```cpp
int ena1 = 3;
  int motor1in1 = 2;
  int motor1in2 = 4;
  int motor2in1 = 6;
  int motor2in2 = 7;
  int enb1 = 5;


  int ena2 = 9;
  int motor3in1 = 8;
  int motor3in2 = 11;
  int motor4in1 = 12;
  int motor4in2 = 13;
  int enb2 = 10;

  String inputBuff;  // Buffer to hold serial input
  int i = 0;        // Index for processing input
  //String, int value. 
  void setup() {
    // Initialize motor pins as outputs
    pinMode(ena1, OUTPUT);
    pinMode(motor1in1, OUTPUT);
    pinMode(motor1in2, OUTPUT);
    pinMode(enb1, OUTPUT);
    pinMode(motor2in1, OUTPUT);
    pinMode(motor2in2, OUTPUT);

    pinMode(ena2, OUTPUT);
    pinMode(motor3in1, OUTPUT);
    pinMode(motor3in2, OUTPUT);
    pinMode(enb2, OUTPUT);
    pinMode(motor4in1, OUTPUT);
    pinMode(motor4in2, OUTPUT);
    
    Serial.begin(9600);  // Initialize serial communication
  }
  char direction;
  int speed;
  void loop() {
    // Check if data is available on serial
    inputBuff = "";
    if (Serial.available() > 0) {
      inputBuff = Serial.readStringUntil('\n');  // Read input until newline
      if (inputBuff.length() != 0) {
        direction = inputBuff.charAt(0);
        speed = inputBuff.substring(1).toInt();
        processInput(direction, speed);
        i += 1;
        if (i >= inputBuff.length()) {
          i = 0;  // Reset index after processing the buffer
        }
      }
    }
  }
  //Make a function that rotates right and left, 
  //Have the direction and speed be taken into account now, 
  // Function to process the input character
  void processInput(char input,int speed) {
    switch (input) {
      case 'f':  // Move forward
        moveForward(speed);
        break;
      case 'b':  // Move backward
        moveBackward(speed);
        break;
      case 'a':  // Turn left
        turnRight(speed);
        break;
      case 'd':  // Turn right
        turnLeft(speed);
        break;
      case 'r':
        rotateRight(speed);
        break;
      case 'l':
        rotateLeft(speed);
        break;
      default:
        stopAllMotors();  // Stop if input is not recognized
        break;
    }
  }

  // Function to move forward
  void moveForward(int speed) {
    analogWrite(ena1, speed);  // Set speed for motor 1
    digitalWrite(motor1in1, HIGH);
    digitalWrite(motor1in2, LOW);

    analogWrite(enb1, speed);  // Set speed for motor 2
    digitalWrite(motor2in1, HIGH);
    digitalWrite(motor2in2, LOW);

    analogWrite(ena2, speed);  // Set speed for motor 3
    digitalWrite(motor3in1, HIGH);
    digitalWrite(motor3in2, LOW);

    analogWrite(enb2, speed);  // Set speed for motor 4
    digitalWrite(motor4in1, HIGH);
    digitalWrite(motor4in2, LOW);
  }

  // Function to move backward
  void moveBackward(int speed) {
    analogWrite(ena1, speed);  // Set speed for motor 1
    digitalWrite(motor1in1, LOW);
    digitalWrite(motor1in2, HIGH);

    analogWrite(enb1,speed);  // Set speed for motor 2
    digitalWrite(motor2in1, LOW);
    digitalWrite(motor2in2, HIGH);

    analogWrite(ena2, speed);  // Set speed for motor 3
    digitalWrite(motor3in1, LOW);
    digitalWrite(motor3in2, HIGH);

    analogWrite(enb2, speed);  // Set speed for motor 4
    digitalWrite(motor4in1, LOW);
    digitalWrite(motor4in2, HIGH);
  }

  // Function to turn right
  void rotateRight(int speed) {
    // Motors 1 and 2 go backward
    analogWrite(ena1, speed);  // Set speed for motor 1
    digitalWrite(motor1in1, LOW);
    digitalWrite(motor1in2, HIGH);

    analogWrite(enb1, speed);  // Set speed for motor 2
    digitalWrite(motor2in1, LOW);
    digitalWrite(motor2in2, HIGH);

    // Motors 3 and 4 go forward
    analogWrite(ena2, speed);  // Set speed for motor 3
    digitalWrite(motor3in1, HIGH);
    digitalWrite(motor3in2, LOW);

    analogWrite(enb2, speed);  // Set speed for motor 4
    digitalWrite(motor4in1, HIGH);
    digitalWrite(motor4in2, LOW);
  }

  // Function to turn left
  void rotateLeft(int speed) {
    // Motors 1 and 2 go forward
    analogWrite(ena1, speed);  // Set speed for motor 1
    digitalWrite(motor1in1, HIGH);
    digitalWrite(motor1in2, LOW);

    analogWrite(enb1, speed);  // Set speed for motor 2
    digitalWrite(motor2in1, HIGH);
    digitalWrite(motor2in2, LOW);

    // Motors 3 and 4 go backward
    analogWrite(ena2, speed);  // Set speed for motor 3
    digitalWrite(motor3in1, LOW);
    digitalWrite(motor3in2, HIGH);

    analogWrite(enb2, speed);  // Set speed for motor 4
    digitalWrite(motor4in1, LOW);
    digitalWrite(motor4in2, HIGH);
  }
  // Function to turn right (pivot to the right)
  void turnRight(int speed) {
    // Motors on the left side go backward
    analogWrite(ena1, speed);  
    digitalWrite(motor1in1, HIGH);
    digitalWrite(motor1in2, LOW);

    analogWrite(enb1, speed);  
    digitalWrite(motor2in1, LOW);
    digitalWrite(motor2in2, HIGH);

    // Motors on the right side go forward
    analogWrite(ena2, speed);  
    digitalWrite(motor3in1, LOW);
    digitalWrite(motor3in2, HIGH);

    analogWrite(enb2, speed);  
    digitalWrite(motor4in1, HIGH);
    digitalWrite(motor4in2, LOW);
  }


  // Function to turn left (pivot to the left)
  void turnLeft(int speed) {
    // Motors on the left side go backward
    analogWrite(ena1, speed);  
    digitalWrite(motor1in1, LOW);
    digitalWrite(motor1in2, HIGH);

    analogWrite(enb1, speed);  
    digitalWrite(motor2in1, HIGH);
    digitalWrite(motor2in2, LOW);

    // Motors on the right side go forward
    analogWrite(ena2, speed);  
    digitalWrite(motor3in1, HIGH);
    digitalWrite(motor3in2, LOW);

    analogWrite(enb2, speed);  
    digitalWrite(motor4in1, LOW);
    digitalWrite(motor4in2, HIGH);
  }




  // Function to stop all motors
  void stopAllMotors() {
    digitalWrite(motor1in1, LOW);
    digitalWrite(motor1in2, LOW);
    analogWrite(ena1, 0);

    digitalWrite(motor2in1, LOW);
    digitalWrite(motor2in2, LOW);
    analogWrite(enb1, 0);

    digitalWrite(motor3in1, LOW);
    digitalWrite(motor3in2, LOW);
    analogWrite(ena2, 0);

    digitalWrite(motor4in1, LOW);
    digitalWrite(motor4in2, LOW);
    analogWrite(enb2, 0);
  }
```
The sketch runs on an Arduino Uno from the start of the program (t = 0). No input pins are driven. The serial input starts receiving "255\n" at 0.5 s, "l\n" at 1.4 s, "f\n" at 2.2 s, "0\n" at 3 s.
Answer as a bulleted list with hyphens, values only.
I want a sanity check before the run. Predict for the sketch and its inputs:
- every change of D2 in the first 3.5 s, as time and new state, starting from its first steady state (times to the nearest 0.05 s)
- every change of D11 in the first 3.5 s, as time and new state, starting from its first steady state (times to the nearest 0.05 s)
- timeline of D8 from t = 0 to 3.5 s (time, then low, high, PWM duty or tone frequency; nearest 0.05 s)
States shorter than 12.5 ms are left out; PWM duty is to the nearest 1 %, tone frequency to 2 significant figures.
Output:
- 0 s low; 1.4 s high; 3 s low
- 0 s low; 1.4 s high; 2.2 s low
- 0 s low; 2.2 s high; 3 s low
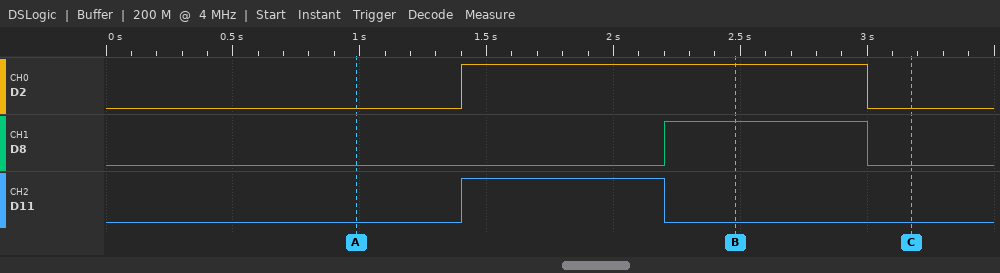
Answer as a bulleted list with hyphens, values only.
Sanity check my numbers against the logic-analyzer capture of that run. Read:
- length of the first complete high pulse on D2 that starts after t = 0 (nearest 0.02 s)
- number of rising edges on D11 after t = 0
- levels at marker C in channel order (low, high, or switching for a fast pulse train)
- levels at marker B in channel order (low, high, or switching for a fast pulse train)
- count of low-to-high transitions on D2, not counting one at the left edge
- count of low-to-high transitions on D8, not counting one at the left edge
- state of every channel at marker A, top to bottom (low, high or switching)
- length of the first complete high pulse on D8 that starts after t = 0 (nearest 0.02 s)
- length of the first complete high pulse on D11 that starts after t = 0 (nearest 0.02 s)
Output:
- 1.60 s
- 1
- D2 low, D8 low, D11 low
- D2 high, D8 high, D11 low
- 1
- 1
- D2 low, D8 low, D11 low
- 0.80 s
- 0.80 s
